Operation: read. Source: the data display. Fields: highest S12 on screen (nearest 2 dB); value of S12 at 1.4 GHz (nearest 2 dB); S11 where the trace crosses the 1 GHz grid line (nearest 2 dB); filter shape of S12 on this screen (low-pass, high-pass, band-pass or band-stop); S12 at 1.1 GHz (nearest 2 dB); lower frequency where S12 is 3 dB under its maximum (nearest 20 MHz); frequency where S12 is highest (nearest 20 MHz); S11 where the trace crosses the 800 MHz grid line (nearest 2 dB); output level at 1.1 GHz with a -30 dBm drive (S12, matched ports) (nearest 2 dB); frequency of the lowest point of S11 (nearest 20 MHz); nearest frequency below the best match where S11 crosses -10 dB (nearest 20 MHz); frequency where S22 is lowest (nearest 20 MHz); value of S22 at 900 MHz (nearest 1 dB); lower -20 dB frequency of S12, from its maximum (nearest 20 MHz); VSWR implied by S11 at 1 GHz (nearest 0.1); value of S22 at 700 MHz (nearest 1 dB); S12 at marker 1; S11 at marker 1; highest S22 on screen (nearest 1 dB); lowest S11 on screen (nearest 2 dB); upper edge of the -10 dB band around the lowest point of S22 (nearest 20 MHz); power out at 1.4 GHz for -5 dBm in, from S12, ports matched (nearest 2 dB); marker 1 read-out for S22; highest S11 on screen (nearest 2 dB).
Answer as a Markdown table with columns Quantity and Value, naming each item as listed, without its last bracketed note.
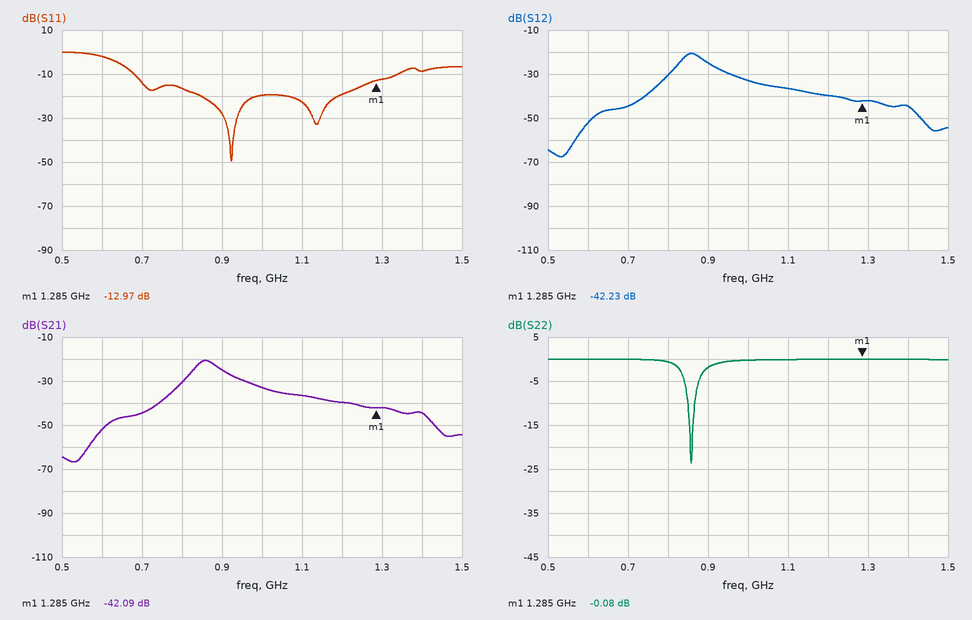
| Quantity | Value |
|---|---|
| highest S12 on screen | -20 dB |
| value of S12 at 1.4 GHz | -44 dB |
| S11 where the trace crosses the 1 GHz grid line | -20 dB |
| filter shape of S12 on this screen | band-pass |
| S12 at 1.1 GHz | -36 dB |
| lower frequency where S12 is 3 dB under its maximum | 840 MHz |
| frequency where S12 is highest | 860 MHz |
| S11 where the trace crosses the 800 MHz grid line | -16 dB |
| output level at 1.1 GHz with a -30 dBm drive (S12, matched ports) | -66 dBm |
| frequency of the lowest point of S11 | 920 MHz |
| nearest frequency below the best match where S11 crosses -10 dB | 680 MHz |
| frequency where S22 is lowest | 860 MHz |
| value of S22 at 900 MHz | -2 dB |
| lower -20 dB frequency of S12, from its maximum | 740 MHz |
| VSWR implied by S11 at 1 GHz | 1.2 |
| value of S22 at 700 MHz | 0 dB |
| S12 at marker 1 | -42.23 dB |
| S11 at marker 1 | -12.97 dB |
| highest S22 on screen | 0 dB |
| lowest S11 on screen | -50 dB |
| upper edge of the -10 dB band around the lowest point of S22 | 860 MHz |
| power out at 1.4 GHz for -5 dBm in, from S12, ports matched | -50 dBm |
| marker 1 read-out for S22 | -0.08 dB |
| highest S11 on screen | 0 dB |
